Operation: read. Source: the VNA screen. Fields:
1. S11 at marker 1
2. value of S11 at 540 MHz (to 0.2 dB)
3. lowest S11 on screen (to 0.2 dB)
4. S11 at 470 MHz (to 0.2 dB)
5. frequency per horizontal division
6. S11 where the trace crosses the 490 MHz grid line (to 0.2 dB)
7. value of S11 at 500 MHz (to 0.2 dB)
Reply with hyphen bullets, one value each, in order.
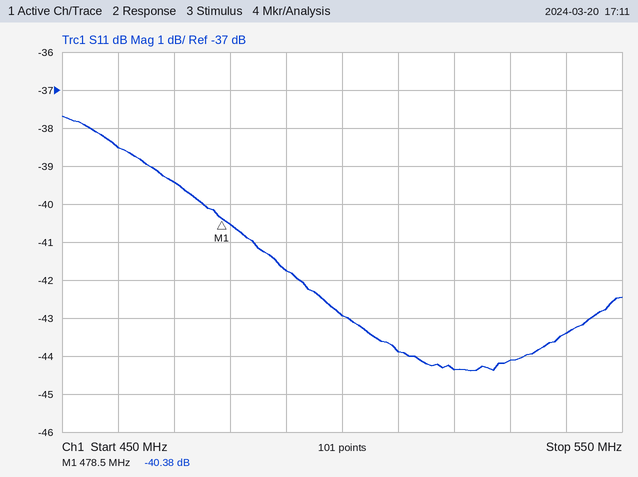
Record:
- -40.38 dB
- -43.4 dB
- -44.4 dB
- -39.4 dB
- 10 MHz
- -41.8 dB
- -43.0 dB
